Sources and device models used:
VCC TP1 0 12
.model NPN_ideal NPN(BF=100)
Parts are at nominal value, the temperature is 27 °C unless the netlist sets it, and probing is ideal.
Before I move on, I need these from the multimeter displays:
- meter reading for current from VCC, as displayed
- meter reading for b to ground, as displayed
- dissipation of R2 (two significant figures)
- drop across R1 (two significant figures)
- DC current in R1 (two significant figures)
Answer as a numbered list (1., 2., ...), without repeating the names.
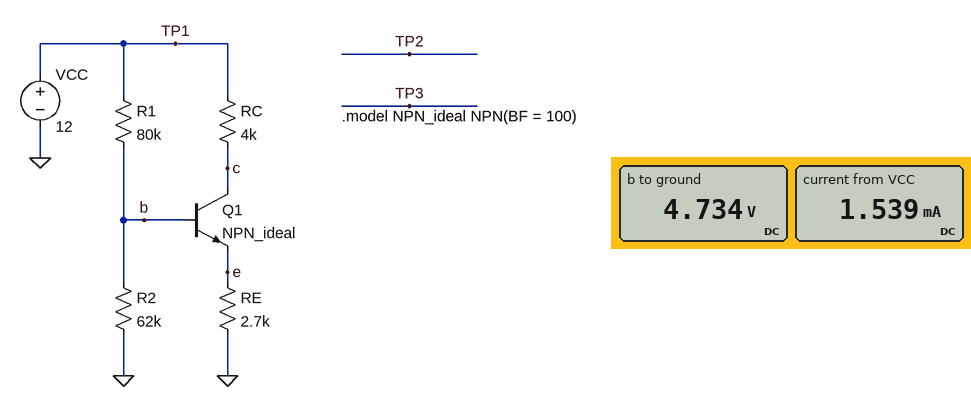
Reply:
1. 1.539 mA
2. 4.734 V
3. 360 µW
4. 7.3 V
5. 91 µA
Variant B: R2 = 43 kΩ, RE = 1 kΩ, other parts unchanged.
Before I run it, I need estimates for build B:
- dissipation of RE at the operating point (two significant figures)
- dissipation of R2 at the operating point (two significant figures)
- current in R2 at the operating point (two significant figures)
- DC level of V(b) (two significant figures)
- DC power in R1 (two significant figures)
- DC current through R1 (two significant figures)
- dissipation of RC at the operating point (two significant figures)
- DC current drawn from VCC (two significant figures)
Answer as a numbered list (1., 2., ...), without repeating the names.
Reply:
1. 5.8 mW
2. 240 µW
3. 74 µA
4. 3.2 V
5. 970 µW
6. 110 µA
7. 22 mW
8. 2.5 mA
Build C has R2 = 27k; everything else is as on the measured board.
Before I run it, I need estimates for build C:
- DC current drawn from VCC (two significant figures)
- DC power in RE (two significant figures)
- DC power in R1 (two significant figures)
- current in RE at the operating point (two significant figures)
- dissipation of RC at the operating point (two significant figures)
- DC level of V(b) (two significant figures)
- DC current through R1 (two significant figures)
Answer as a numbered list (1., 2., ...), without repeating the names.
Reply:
1. 890 µA
2. 1.6 mW
3. 1.0 mW
4. 780 µA
5. 2.4 mW
6. 2.9 V
7. 110 µA
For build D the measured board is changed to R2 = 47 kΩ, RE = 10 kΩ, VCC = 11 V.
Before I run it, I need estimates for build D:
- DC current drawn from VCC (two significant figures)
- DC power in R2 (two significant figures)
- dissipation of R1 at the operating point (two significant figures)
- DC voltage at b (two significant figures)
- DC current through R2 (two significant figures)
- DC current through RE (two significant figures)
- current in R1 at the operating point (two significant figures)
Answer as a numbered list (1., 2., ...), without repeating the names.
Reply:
1. 410 µA
2. 340 µW
3. 620 µW
4. 4.0 V
5. 85 µA
6. 320 µA
7. 88 µA
